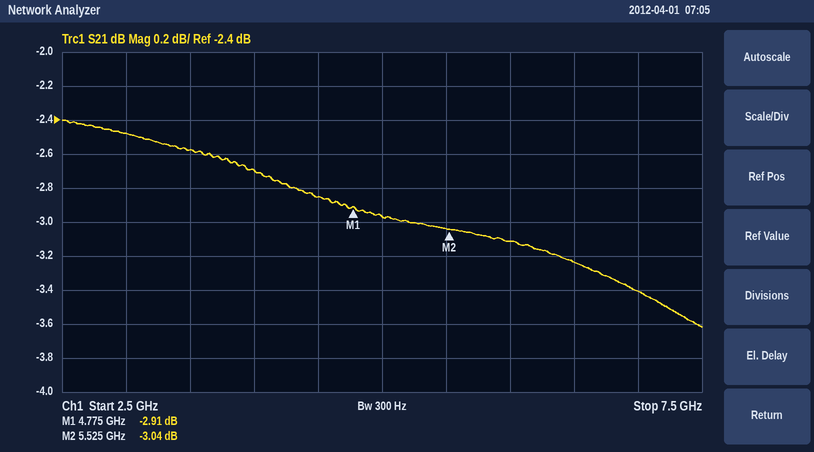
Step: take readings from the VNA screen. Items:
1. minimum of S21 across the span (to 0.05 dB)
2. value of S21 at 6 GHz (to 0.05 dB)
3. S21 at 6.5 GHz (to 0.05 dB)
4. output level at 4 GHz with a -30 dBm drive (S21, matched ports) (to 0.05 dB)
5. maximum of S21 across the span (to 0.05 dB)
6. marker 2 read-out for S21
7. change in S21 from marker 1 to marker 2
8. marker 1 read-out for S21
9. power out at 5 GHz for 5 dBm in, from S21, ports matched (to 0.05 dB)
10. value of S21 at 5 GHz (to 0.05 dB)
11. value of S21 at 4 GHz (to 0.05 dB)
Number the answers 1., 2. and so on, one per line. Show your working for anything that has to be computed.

1. -3.60 dB
2. -3.10 dB
3. -3.25 dB
4. -30 dBm + (-2.70 dB) = -32.70 dBm
5. -2.40 dB
6. -3.04 dB
7. -3.04 − (-2.91) = -0.13 dB
8. -2.91 dB
9. 5 dBm + (-2.95 dB) = 2.05 dBm
10. -2.95 dB
11. -2.70 dB
